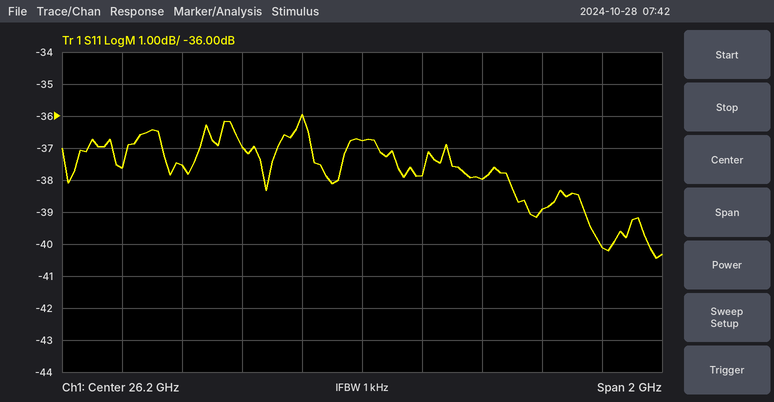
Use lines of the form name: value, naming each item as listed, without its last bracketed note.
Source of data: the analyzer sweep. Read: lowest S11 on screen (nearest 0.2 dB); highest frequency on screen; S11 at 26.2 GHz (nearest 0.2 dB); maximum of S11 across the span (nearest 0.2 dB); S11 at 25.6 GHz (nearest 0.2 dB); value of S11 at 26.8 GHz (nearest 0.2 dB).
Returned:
lowest S11 on screen: -40.4 dB
highest frequency on screen: 27.2 GHz
S11 at 26.2 GHz: -36.8 dB
maximum of S11 across the span: -36.0 dB
S11 at 25.6 GHz: -37.6 dB
value of S11 at 26.8 GHz: -39.0 dB
